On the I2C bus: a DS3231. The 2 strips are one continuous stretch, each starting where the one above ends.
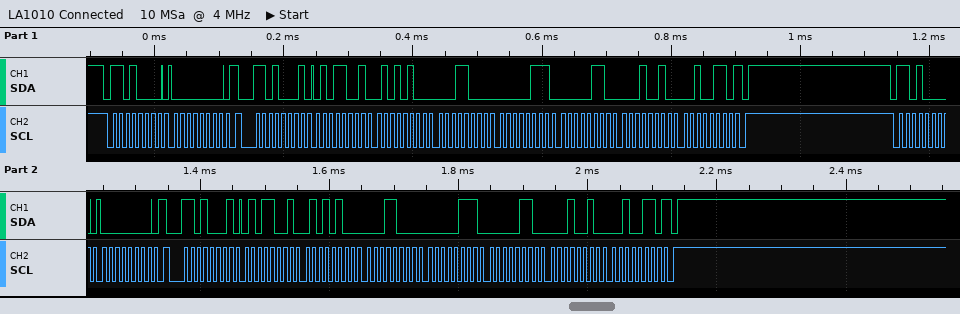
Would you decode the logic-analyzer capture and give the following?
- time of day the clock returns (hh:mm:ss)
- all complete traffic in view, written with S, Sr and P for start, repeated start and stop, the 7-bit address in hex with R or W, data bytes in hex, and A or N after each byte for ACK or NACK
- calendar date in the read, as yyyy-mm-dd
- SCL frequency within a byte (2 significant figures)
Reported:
18:54:59
S 68W A 00 A Sr 68R A 59 A 54 A 18 A 07 A 06 A 12 A 26 N P S 68W A 00 A Sr 68R A 59 A 54 A 18 A 07 A 06 A 12 A 26 N P
2026-12-06
100 kHz
